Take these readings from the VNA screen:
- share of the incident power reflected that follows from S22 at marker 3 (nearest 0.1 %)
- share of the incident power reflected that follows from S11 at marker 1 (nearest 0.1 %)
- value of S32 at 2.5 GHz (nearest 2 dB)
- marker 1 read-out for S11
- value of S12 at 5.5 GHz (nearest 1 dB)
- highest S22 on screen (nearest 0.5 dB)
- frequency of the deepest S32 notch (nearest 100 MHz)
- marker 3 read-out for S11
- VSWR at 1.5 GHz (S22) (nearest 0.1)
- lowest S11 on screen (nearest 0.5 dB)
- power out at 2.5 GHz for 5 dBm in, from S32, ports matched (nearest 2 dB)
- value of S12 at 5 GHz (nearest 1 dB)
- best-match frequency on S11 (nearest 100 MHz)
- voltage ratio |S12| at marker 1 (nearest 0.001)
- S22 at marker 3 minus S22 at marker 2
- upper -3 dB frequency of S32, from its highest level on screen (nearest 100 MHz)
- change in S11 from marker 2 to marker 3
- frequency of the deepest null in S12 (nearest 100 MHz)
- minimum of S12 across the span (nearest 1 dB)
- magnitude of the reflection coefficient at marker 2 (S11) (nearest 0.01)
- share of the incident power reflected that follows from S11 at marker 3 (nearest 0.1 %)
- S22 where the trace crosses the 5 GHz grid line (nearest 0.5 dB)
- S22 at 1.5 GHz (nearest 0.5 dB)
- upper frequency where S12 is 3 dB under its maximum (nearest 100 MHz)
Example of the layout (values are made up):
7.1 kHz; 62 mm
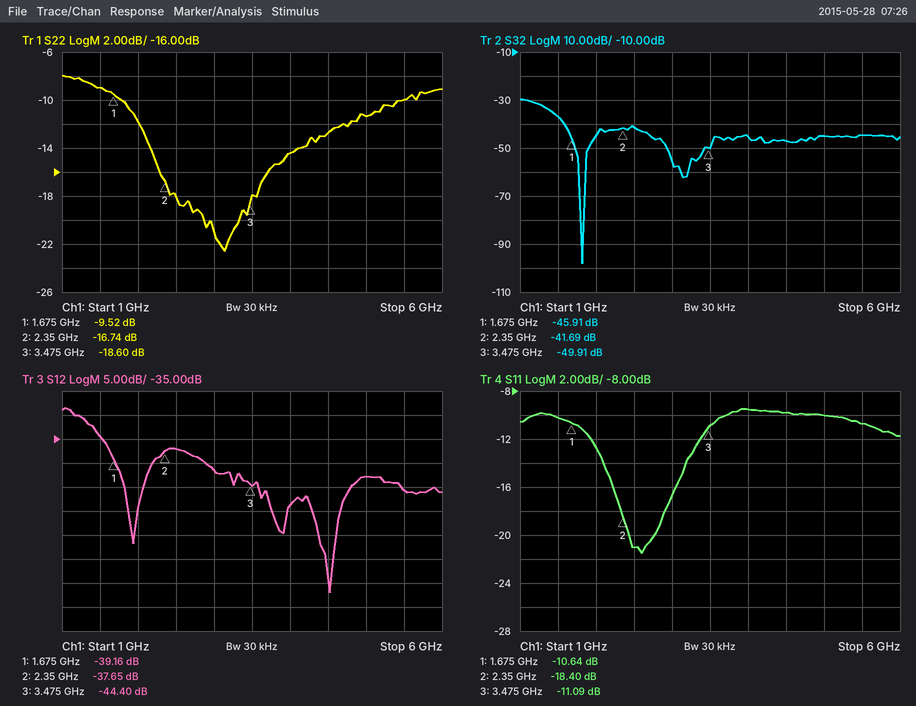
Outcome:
1.4 %; 8.6 %; -42 dB; -10.64 dB; -46 dB; -8.0 dB; 1.8 GHz; -11.09 dB; 2.1; -21.5 dB; -36 dBm; -43 dB; 2.6 GHz; 0.011; -1.86 dB; 1.3 GHz; 7.31 dB; 4.5 GHz; -67 dB; 0.12; 7.8 %; -11.5 dB; -9.0 dB; 1.3 GHz
